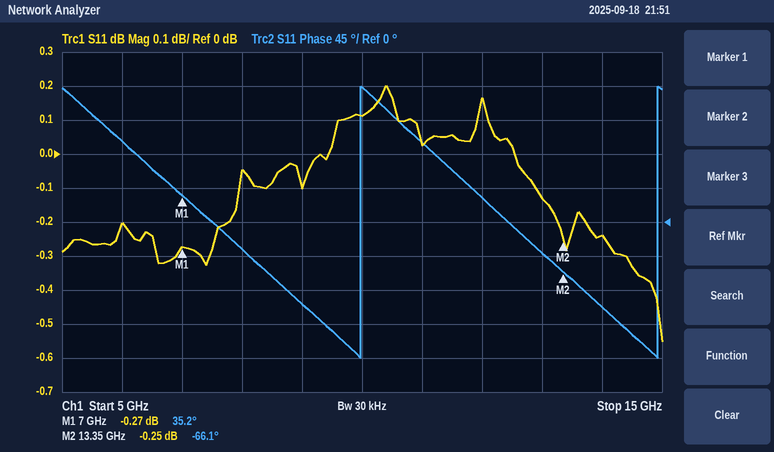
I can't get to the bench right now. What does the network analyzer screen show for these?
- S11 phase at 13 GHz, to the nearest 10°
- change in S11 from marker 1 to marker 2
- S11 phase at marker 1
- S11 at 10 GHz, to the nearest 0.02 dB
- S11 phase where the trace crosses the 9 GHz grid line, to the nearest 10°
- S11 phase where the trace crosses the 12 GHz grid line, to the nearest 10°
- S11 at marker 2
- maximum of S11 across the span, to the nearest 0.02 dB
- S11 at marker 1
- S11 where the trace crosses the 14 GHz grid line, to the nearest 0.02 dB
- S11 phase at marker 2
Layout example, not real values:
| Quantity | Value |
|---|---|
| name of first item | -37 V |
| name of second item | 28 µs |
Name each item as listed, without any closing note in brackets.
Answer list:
| Quantity | Value |
|---|---|
| S11 phase at 13 GHz, to the nearest 10° | -40° |
| change in S11 from marker 1 to marker 2 | 0.02 dB |
| S11 phase at marker 1 | 35.2° |
| S11 at 10 GHz, to the nearest 0.02 dB | 0.12 dB |
| S11 phase where the trace crosses the 9 GHz grid line, to the nearest 10° | -110° |
| S11 phase where the trace crosses the 12 GHz grid line, to the nearest 10° | 30° |
| S11 at marker 2 | -0.25 dB |
| maximum of S11 across the span, to the nearest 0.02 dB | 0.20 dB |
| S11 at marker 1 | -0.27 dB |
| S11 where the trace crosses the 14 GHz grid line, to the nearest 0.02 dB | -0.24 dB |
| S11 phase at marker 2 | -66.1° |
